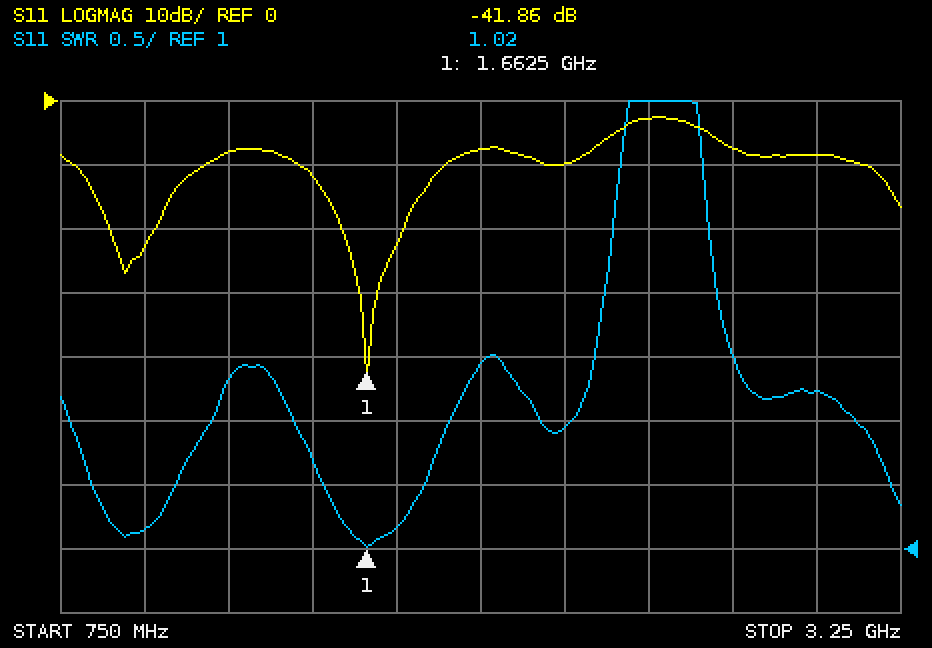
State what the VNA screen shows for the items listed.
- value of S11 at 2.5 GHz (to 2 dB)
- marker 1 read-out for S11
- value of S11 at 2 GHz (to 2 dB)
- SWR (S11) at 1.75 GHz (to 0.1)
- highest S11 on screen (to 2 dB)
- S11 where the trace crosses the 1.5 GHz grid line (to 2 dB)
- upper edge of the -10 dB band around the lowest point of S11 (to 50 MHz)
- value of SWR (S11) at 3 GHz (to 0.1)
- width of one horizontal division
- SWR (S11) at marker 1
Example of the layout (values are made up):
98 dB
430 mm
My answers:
-2 dB
-41.86 dB
-8 dB
1.2
-2 dB
-12 dB
1.90 GHz
2.2
250 MHz
1.02
